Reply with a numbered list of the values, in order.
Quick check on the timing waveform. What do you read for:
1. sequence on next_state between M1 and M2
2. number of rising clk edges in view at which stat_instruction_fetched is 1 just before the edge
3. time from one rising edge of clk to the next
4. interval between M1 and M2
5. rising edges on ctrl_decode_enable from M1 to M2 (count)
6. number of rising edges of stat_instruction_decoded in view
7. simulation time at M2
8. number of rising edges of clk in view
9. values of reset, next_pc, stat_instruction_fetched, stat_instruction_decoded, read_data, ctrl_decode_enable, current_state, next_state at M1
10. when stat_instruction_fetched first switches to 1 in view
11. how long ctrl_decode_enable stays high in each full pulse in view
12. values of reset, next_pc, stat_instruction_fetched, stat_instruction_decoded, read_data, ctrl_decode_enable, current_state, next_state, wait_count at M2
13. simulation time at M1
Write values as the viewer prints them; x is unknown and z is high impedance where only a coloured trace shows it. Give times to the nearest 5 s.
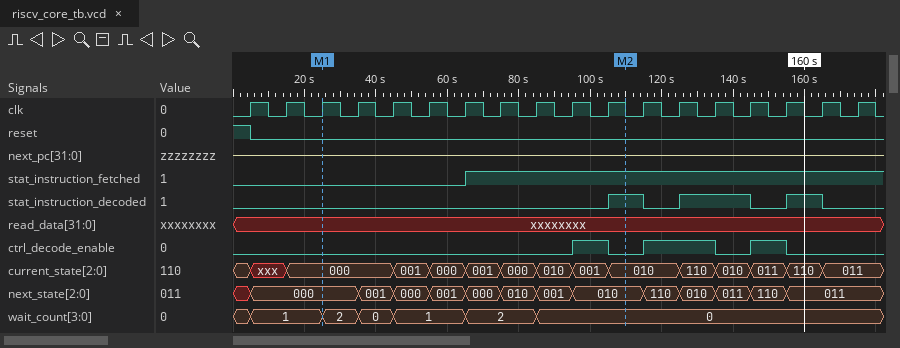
1. 000, 001, 000, 001, 000, 010, 001, 010
2. 11
3. 10 s
4. 85 s
5. 1
6. 3
7. 110 s
8. 18
9. reset=0, next_pc=z, stat_instruction_fetched=0, stat_instruction_decoded=0, read_data=xxxxxxxx, ctrl_decode_enable=0, current_state=000, next_state=000
10. 65 s
11. 10 s, 20 s, 10 s
12. reset=0, next_pc=z, stat_instruction_fetched=1, stat_instruction_decoded=1, read_data=xxxxxxxx, ctrl_decode_enable=0, current_state=010, next_state=010, wait_count=0
13. 25 s
